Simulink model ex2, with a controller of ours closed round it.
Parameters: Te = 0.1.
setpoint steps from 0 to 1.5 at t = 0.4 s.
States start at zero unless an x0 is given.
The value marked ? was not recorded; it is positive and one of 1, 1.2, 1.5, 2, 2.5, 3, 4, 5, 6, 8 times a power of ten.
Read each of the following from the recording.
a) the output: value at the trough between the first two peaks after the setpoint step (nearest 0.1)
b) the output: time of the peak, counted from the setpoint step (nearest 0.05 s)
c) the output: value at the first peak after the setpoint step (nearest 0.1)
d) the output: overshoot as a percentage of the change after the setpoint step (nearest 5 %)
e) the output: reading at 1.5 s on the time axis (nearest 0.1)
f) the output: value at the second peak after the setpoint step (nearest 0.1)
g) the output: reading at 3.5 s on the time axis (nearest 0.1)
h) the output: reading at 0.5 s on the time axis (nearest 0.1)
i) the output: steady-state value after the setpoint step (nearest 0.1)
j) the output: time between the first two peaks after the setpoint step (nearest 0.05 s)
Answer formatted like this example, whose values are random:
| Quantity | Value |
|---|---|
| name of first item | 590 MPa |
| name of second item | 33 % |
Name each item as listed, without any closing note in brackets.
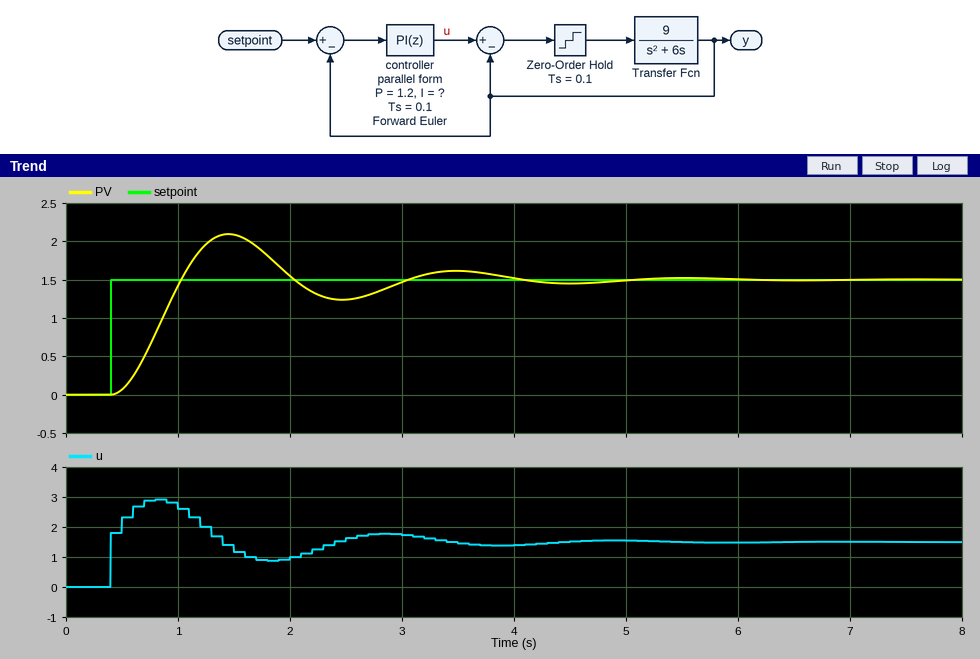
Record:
| Quantity | Value |
|---|---|
| the output: value at the trough between the first two peaks after the setpoint step | 1.2 |
| the output: time of the peak, counted from the setpoint step | 1.05 s |
| the output: value at the first peak after the setpoint step | 2.1 |
| the output: overshoot as a percentage of the change after the setpoint step | 40 % |
| the output: reading at 1.5 s on the time axis | 2.1 |
| the output: value at the second peak after the setpoint step | 1.6 |
| the output: reading at 3.5 s on the time axis | 1.6 |
| the output: reading at 0.5 s on the time axis | 0.1 |
| the output: steady-state value after the setpoint step | 1.5 |
| the output: time between the first two peaks after the setpoint step | 2.05 s |
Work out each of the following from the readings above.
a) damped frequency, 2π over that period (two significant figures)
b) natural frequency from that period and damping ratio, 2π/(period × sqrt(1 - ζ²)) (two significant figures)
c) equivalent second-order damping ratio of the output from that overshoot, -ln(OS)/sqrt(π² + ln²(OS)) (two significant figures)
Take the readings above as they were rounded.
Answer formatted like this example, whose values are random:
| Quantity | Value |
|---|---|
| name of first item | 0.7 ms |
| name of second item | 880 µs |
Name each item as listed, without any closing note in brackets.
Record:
| Quantity | Value |
|---|---|
| damped frequency, 2π over that period | 3.1 rad/s |
| natural frequency from that period and damping ratio, 2π/(period × sqrt(1 - ζ²)) | 3.2 rad/s |
| equivalent second-order damping ratio of the output from that overshoot, -ln(OS)/sqrt(π² + ln²(OS)) | 0.28 |
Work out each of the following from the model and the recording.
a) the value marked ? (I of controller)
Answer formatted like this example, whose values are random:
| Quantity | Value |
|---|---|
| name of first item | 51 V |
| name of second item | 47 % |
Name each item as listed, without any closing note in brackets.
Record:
| Quantity | Value |
|---|---|
| the value marked ? | 4 |
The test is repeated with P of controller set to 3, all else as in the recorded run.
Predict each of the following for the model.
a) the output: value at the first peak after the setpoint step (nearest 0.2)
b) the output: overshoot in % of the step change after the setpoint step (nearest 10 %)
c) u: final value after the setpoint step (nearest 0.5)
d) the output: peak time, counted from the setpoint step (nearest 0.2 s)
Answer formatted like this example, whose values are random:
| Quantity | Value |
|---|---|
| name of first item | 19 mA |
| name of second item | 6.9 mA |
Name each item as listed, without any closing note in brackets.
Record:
| Quantity | Value |
|---|---|
| the output: value at the first peak after the setpoint step | 2.0 |
| the output: overshoot in % of the step change after the setpoint step | 30 % |
| u: final value after the setpoint step | 1.5 |
| the output: peak time, counted from the setpoint step | 0.6 s |
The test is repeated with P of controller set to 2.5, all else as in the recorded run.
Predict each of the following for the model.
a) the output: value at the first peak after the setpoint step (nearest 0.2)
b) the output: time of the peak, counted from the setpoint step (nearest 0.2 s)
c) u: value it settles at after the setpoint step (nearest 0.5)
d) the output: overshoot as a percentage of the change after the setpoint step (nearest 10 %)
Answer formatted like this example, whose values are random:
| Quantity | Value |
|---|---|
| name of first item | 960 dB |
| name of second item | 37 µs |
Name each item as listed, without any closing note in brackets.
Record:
| Quantity | Value |
|---|---|
| the output: value at the first peak after the setpoint step | 2.0 |
| the output: time of the peak, counted from the setpoint step | 0.8 s |
| u: value it settles at after the setpoint step | 1.5 |
| the output: overshoot as a percentage of the change after the setpoint step | 30 % |
